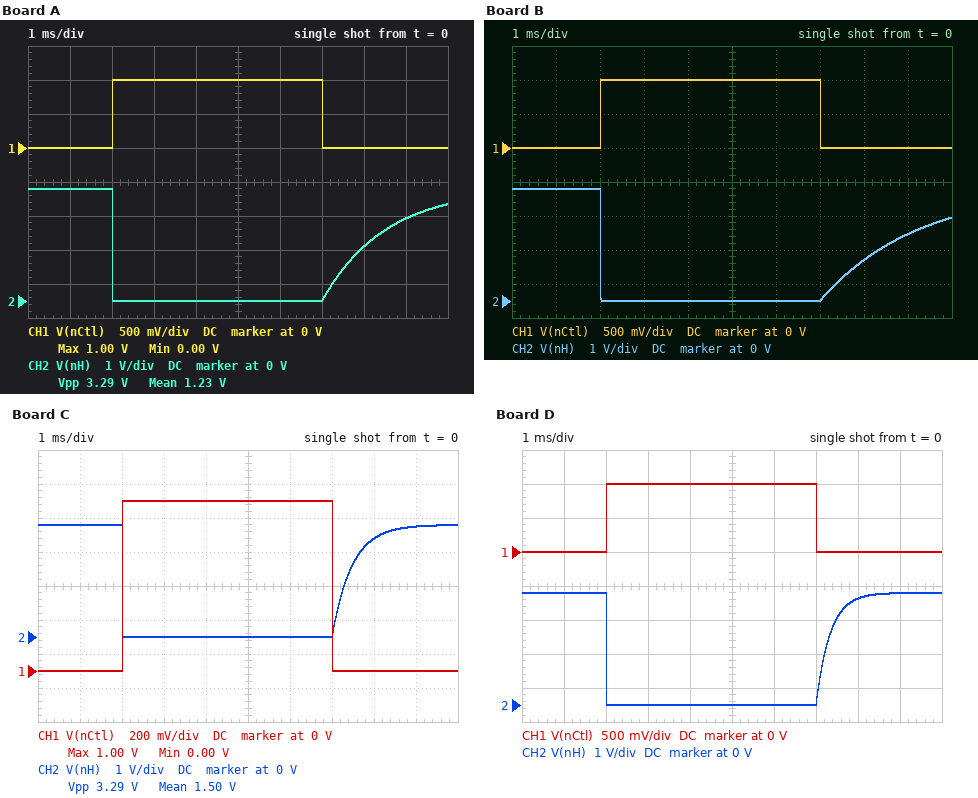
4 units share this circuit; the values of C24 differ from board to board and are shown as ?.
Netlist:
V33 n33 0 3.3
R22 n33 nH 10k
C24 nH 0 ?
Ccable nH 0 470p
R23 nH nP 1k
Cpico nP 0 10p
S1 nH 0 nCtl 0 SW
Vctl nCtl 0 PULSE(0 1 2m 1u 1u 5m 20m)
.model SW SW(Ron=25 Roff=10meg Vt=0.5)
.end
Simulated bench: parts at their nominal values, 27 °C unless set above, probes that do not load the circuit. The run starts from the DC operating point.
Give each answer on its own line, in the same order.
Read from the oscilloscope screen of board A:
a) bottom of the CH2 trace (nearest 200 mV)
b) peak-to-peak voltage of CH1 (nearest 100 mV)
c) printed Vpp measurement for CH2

0 V
1.0 V
3.29 V
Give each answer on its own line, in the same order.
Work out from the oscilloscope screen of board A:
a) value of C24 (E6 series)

150 nF
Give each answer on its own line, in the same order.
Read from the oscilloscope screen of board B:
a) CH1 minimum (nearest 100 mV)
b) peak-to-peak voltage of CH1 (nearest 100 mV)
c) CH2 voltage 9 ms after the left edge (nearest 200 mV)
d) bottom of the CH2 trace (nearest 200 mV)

0 V
1.0 V
2.0 V
0 V
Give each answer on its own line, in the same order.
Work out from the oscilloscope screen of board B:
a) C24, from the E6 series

220 nF
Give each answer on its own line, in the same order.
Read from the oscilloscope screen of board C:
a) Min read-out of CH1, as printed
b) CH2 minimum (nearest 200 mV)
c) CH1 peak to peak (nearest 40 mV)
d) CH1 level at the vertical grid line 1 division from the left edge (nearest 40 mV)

0.00 V
0 V
1.00 V
0 V
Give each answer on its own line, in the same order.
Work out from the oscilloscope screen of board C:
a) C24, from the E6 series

47 nF
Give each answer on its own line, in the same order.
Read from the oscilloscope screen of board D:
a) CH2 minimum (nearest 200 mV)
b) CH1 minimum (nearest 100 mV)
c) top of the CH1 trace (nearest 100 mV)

0 V
0 V
1.0 V
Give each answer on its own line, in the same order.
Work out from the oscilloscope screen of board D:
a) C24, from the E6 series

33 nF
